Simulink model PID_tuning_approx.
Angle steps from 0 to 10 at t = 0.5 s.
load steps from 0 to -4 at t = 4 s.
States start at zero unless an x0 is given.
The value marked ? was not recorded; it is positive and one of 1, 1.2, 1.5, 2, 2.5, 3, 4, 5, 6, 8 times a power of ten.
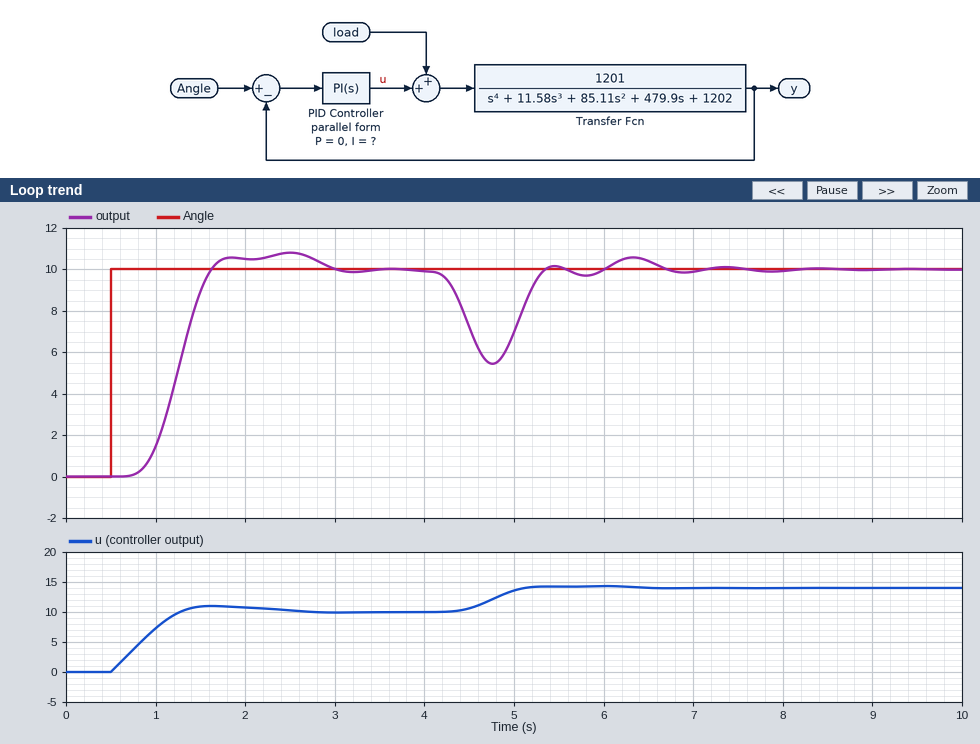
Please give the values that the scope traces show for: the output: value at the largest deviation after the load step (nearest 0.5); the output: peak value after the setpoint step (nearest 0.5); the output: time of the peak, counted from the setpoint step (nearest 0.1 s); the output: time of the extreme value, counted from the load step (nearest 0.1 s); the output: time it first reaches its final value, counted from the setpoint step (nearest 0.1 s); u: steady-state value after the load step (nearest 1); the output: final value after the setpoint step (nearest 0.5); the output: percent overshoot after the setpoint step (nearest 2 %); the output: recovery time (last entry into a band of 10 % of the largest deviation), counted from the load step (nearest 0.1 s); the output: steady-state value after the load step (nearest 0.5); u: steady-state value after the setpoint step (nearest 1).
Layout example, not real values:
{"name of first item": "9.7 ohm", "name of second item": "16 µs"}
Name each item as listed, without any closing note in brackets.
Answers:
{"the output: value at the largest deviation after the load step": "5.5", "the output: peak value after the setpoint step": "11.0", "the output: time of the peak, counted from the setpoint step": "2.0 s", "the output: time of the extreme value, counted from the load step": "0.8 s", "the output: time it first reaches its final value, counted from the setpoint step": "1.1 s", "u: steady-state value after the load step": "14", "the output: final value after the setpoint step": "10.0", "the output: percent overshoot after the setpoint step": "8 %", "the output: recovery time (last entry into a band of 10 % of the largest deviation), counted from the load step": "2.5 s", "the output: steady-state value after the load step": "10.0", "u: steady-state value after the setpoint step": "10"}
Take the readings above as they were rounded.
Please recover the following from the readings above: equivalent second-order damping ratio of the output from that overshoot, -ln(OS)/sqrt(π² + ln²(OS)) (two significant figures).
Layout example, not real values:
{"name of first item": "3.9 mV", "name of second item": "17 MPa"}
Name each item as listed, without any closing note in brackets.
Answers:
{"equivalent second-order damping ratio of the output from that overshoot, -ln(OS)/sqrt(π² + ln²(OS))": "0.63"}
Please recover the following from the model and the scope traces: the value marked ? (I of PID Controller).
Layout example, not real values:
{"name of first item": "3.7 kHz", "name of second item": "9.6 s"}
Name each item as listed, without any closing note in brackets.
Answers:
{"the value marked ?": "1.5"}
